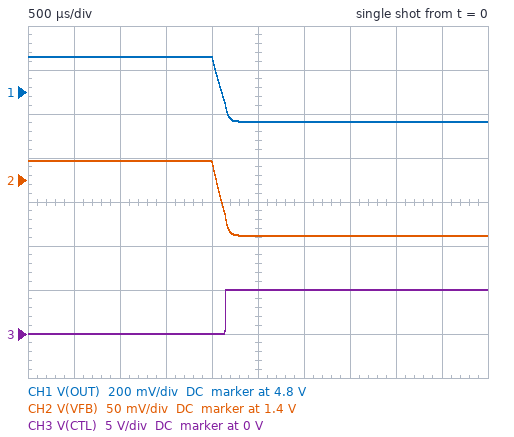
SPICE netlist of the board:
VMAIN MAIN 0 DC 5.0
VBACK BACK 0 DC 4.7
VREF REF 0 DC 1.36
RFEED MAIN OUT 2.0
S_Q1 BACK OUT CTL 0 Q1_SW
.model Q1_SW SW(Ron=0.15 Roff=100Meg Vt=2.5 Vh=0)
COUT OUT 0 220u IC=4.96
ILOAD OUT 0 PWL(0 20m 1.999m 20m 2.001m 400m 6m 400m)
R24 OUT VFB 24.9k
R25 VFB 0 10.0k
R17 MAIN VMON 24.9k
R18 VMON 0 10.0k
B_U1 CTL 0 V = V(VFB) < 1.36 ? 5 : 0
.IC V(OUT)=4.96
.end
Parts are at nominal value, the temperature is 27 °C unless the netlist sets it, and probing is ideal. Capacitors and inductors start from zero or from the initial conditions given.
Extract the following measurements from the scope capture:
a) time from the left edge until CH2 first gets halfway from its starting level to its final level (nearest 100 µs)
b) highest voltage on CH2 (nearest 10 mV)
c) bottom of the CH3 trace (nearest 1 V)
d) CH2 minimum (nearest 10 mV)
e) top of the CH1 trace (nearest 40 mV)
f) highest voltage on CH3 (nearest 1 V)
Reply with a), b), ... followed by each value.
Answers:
a) 2.1 ms
b) 1.42 V
c) 0 V
d) 1.34 V
e) 4.96 V
f) 5 V
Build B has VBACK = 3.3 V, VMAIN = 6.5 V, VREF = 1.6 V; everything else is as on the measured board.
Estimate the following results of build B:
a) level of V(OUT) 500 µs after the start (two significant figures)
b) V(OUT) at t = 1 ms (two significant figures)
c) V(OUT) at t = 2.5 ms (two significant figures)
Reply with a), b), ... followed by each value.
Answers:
a) 6.0 V
b) 6.3 V
c) 5.9 V
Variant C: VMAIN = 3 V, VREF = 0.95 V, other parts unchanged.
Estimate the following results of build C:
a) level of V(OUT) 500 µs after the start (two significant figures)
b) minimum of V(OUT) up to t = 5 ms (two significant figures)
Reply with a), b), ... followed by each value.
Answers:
a) 4.6 V
b) 4.5 V
